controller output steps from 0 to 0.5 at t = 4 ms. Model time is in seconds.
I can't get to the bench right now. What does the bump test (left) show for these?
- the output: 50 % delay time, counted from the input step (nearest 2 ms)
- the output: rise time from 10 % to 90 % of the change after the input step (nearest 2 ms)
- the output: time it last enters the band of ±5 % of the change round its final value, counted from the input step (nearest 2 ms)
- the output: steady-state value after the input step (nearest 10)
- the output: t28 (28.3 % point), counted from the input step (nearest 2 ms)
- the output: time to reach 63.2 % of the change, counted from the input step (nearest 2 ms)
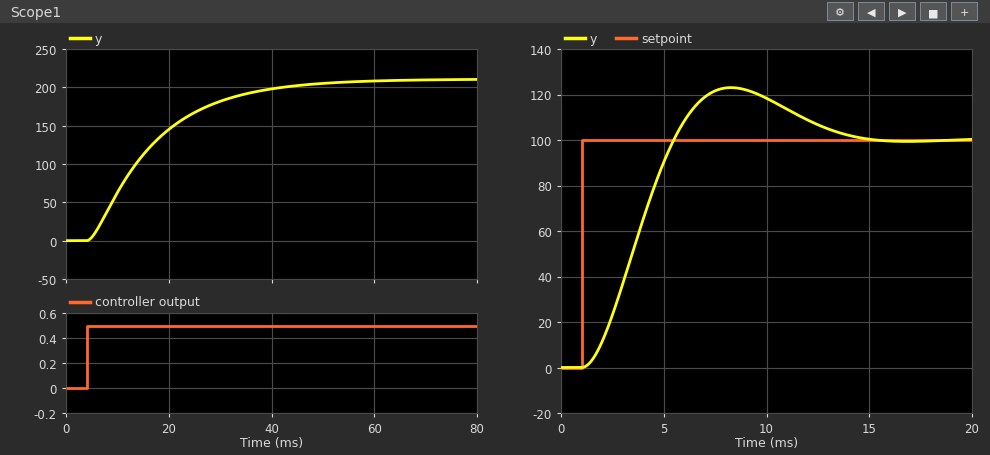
10 ms
28 ms
38 ms
210
6 ms
14 ms
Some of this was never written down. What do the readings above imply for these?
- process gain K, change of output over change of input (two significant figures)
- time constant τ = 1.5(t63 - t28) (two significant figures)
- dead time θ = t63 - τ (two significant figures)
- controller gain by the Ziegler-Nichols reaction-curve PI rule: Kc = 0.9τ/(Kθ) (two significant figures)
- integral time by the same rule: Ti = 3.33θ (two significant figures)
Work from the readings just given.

420
12 ms
2.0 ms
0.013
6.7 ms
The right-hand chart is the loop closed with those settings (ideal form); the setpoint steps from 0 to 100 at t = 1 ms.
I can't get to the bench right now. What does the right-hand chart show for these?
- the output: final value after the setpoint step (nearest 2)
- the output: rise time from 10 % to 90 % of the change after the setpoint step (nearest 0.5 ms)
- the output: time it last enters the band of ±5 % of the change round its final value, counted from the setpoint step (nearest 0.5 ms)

100
3.0 ms
12.0 ms
